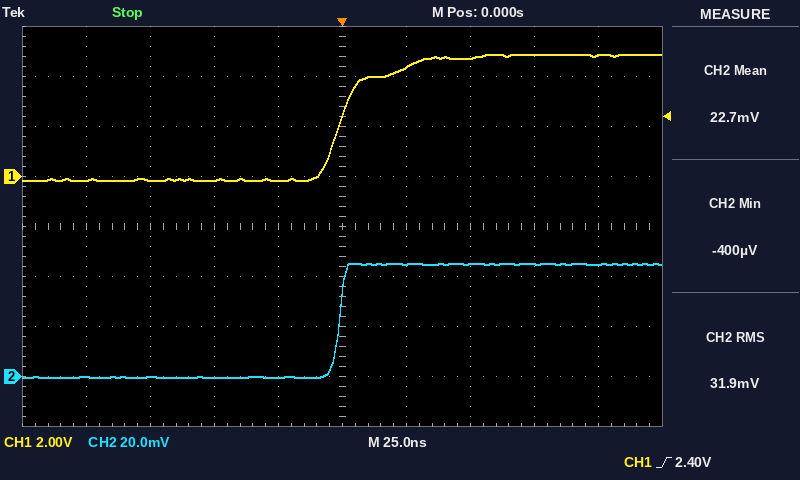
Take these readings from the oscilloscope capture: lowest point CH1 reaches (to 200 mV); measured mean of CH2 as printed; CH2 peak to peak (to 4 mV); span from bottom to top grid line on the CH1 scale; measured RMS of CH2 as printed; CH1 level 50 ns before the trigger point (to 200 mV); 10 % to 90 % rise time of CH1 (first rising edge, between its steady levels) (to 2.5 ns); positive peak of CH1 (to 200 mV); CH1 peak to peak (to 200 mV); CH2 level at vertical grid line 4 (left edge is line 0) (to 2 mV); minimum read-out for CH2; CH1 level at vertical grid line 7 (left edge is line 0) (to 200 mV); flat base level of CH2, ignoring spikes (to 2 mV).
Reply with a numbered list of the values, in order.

1. -200 mV
2. 22.7 mV
3. 44 mV
4. 16 V
5. 31.9 mV
6. -200 mV
7. 32.5 ns
8. 4.8 V
9. 5.0 V
10. 0 mV
11. -400 µV
12. 4.8 V
13. 0 mV
